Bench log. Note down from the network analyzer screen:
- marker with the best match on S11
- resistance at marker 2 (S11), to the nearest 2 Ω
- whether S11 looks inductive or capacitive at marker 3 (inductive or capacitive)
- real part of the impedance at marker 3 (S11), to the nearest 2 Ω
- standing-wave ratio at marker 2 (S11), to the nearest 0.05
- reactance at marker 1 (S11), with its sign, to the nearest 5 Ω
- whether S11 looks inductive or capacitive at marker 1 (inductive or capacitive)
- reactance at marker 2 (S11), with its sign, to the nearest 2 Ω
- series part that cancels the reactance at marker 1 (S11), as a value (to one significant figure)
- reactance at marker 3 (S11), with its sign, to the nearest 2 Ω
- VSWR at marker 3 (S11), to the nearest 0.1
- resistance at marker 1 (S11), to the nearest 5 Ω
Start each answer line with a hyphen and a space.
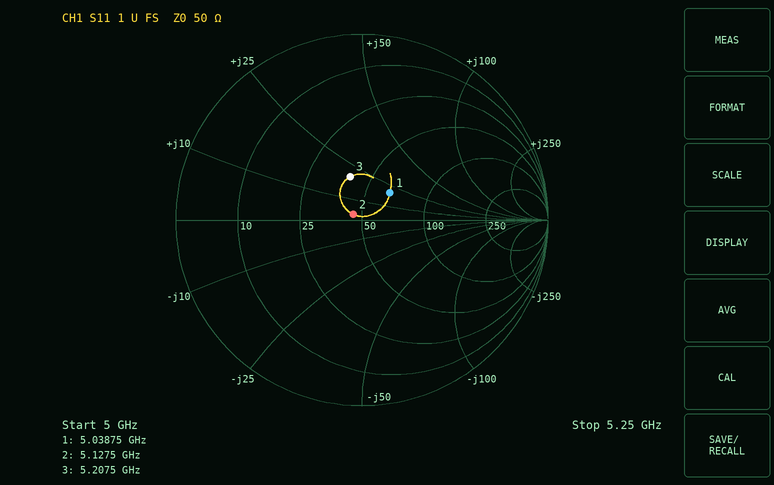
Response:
- marker 2
- 46 Ω
- inductive
- 40 Ω
- 1.10
- +20 Ω
- inductive
- +2 Ω
- 2 pF
- +20 Ω
- 1.6
- 65 Ω
